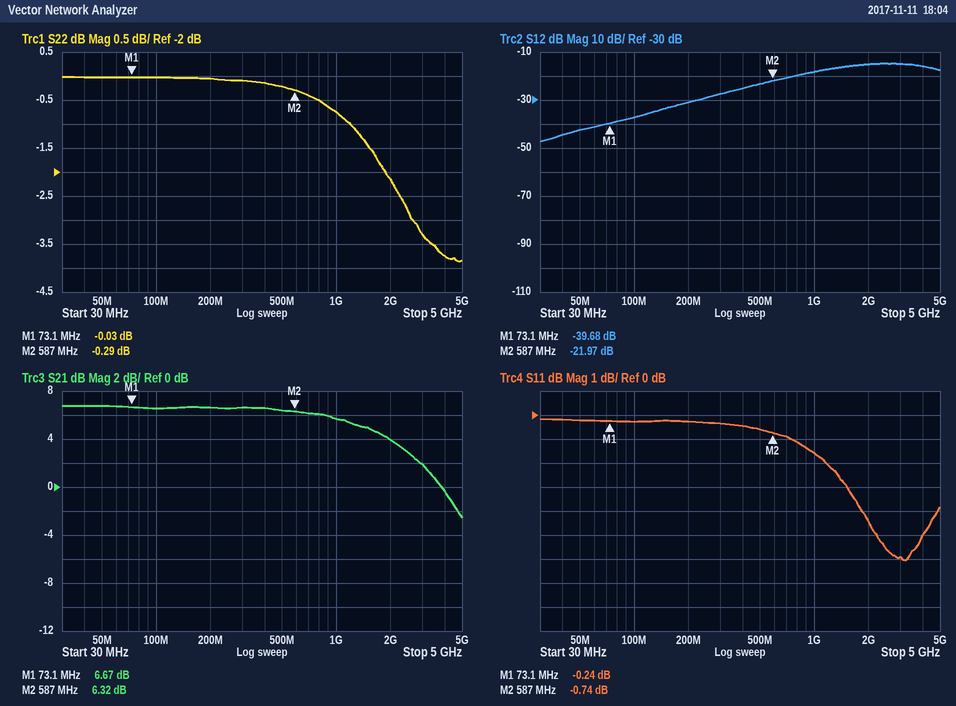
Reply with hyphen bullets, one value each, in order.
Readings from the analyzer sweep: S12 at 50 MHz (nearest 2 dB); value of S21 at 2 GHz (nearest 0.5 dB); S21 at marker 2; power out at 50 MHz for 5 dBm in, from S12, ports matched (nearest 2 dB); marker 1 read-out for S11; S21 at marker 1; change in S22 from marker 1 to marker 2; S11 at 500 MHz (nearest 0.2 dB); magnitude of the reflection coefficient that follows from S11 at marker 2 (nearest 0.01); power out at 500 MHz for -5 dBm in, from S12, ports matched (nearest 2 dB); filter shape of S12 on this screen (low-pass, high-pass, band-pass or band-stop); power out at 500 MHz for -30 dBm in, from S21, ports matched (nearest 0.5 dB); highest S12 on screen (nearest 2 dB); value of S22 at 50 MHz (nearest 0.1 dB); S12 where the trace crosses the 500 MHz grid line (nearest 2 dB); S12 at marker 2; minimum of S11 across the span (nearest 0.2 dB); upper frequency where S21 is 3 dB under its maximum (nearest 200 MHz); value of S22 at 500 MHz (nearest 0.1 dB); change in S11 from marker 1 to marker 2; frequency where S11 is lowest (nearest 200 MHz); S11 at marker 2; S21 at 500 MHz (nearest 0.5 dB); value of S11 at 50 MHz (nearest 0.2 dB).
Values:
- -42 dB
- 4.0 dB
- 6.32 dB
- -38 dBm
- -0.24 dB
- 6.67 dB
- -0.26 dB
- -0.6 dB
- 0.92
- -28 dBm
- high-pass
- -23.5 dBm
- -14 dB
- 0.0 dB
- -24 dB
- -21.97 dB
- -6.0 dB
- 2.0 GHz
- -0.2 dB
- -0.50 dB
- 3.2 GHz
- -0.74 dB
- 6.5 dB
- -0.2 dB
